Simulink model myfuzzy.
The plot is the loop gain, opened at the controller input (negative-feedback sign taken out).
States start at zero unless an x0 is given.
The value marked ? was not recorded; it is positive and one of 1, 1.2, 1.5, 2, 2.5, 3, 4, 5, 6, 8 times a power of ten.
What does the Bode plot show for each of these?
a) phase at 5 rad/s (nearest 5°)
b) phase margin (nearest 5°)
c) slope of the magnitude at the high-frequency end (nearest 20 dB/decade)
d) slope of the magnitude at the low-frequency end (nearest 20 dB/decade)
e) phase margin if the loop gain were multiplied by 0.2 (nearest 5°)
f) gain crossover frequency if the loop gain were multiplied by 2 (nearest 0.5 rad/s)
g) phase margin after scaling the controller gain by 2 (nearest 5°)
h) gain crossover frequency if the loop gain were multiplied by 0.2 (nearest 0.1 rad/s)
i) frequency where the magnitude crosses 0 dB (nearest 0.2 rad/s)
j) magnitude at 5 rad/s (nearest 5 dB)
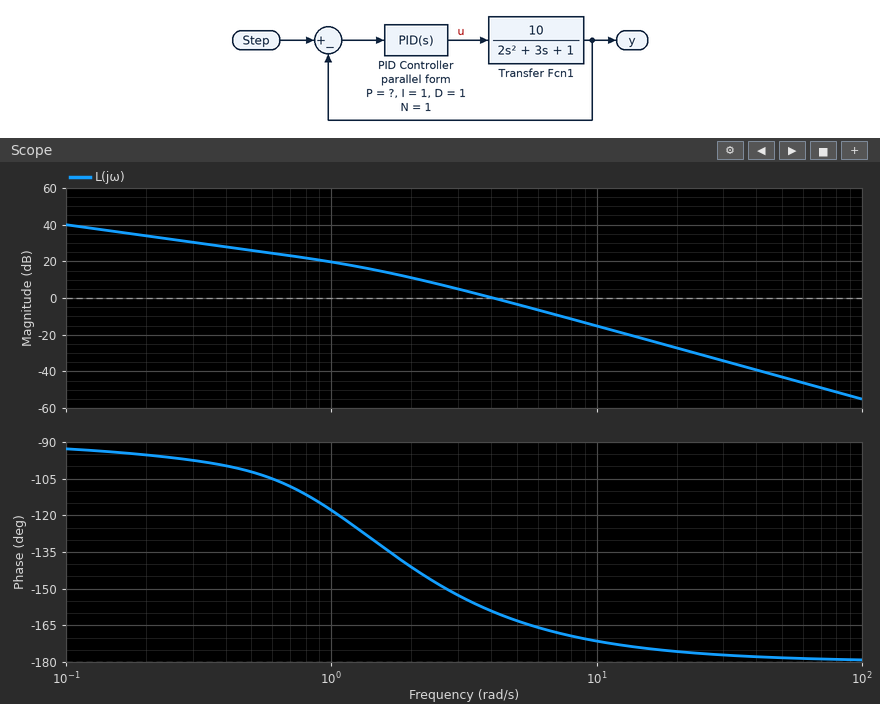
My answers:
-165°
20°
-40 dB/decade
-20 dB/decade
45°
6.0 rad/s
15°
1.6 rad/s
4.0 rad/s
-5 dB
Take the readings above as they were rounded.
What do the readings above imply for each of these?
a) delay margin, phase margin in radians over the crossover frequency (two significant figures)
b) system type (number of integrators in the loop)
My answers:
0.087 s
1
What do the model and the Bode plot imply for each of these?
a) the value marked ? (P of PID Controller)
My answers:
2.5
